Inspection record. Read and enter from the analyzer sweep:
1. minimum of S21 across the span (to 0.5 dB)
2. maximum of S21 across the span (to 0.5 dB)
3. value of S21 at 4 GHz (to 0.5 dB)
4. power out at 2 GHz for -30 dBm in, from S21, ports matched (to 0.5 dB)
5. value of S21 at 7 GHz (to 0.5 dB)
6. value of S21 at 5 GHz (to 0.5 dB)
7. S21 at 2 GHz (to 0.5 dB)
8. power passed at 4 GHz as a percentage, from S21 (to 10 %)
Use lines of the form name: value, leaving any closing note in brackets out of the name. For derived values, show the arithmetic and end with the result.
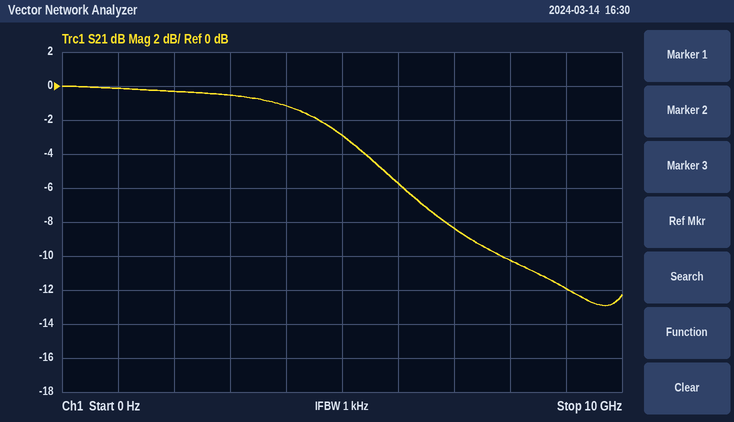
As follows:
minimum of S21 across the span: -13.0 dB
maximum of S21 across the span: 0.0 dB
value of S21 at 4 GHz: -1.0 dB
power out at 2 GHz for -30 dBm in, from S21, ports matched: -30 dBm + (-0.5 dB) = -30.5 dBm
value of S21 at 7 GHz: -8.5 dB
value of S21 at 5 GHz: -3.0 dB
S21 at 2 GHz: -0.5 dB
power passed at 4 GHz as a percentage, from S21: 10^(-1/10) ≈ 79.4 %, so 80 % to the nearest 10 %
